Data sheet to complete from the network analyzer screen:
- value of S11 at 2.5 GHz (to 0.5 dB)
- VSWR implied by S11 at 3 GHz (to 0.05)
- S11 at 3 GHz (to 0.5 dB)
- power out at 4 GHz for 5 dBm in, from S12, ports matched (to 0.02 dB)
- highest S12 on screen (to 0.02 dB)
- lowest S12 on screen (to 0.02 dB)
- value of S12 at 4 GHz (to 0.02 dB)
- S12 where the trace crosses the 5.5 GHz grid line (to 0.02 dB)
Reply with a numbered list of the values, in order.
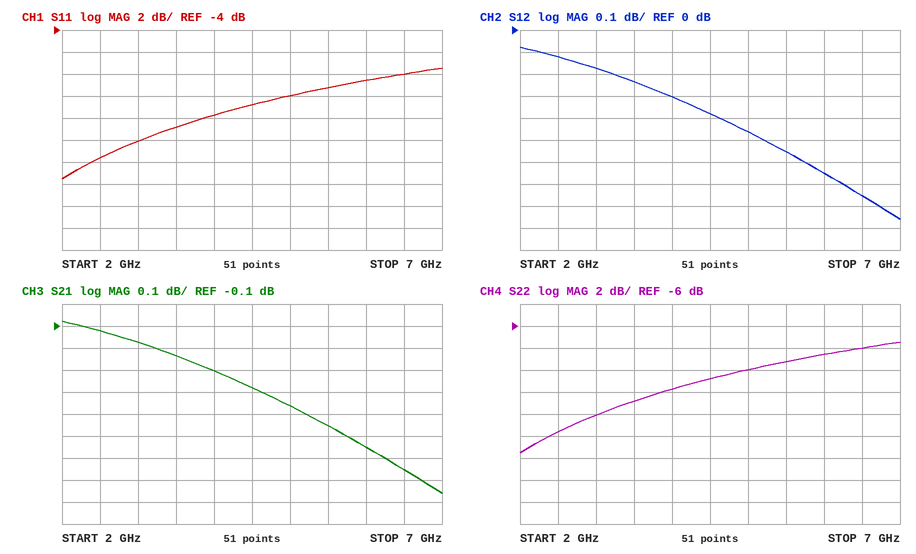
1. -15.5 dB
2. 1.50
3. -14.0 dB
4. 4.70 dBm
5. -0.08 dB
6. -0.86 dB
7. -0.30 dB
8. -0.56 dB
